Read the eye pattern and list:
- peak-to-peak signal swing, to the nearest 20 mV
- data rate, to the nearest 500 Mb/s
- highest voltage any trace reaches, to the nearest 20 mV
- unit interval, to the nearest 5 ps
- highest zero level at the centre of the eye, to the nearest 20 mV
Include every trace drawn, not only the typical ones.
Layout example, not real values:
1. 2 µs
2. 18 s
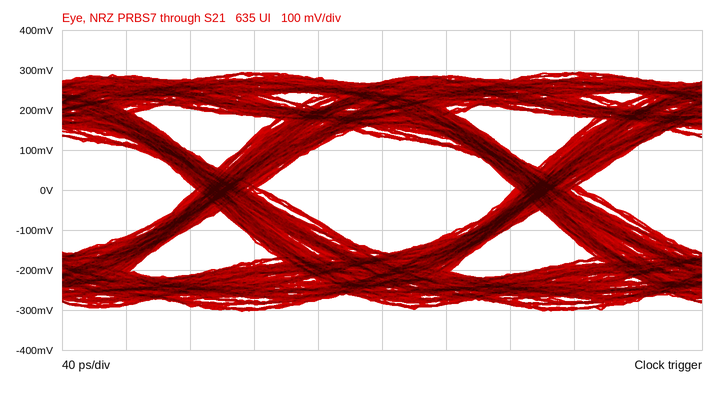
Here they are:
1. 600 mV
2. 5.0 Gb/s
3. 300 mV
4. 200 ps
5. -160 mV
